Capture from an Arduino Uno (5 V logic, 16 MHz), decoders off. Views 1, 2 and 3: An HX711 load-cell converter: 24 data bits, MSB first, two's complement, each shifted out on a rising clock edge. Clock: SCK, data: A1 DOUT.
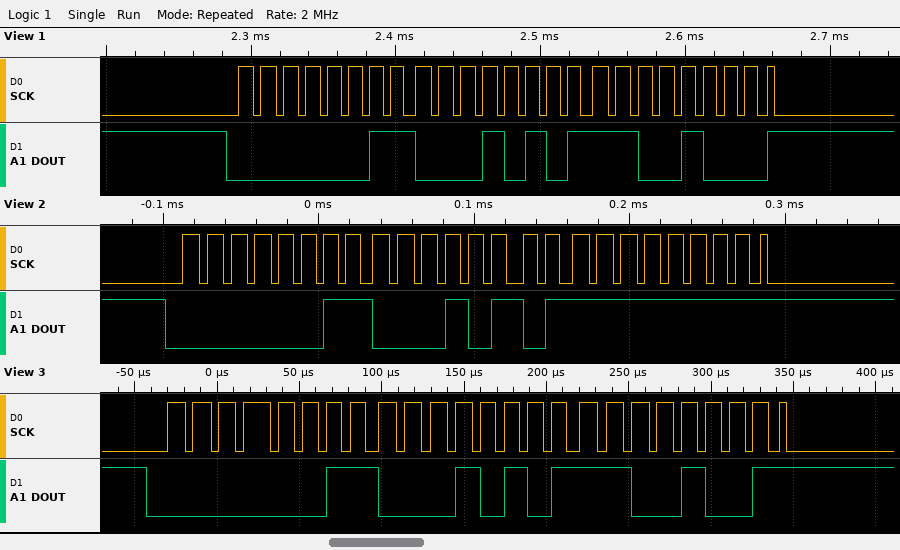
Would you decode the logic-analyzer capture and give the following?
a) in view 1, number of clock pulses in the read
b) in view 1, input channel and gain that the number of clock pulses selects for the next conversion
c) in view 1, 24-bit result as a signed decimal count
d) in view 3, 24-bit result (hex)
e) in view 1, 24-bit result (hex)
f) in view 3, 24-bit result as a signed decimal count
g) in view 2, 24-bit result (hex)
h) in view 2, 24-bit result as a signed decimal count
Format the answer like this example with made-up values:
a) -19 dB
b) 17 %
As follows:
a) 25
b) channel A, gain 128
c) 202184
d) 0x0315C9
e) 0x0315C8
f) 202185
g) 0x0315FF
h) 202239
